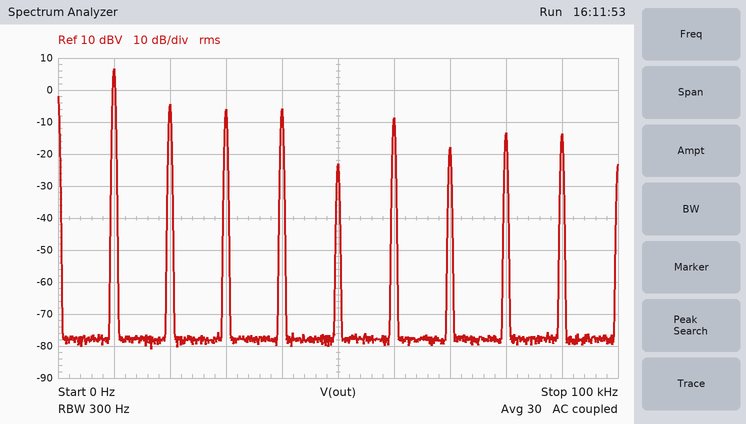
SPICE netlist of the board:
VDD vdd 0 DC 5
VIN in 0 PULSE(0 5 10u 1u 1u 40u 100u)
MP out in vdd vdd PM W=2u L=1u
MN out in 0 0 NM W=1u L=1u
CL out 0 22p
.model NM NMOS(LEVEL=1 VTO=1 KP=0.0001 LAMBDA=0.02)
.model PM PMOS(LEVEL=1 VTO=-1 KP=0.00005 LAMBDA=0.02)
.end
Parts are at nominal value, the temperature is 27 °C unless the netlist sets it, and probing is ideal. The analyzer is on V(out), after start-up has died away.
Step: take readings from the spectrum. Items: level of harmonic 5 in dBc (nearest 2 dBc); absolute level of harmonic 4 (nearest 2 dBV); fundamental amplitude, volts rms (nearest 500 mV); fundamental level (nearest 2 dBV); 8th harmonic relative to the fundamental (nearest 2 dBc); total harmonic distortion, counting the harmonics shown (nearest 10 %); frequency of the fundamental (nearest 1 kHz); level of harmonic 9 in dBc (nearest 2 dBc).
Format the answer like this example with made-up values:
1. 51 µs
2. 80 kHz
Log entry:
1. -30 dBc
2. -6 dBV
3. 2.0 V
4. 6 dBV
5. -20 dBc
6. 50 %
7. 10 kHz
8. -20 dBc
